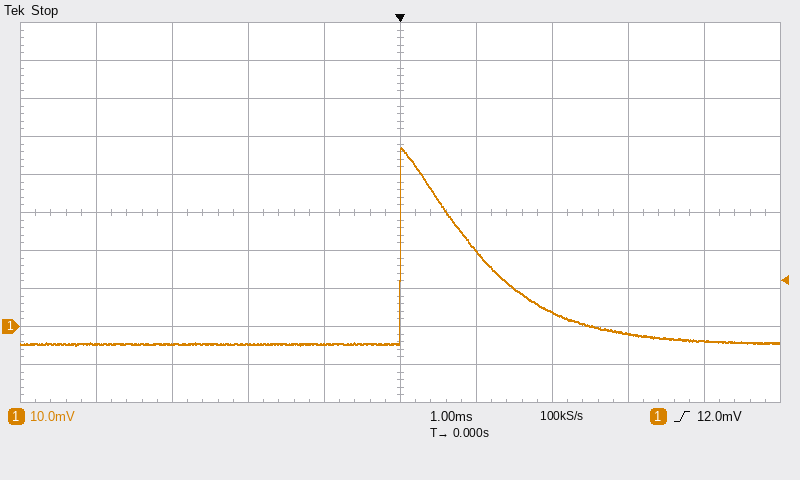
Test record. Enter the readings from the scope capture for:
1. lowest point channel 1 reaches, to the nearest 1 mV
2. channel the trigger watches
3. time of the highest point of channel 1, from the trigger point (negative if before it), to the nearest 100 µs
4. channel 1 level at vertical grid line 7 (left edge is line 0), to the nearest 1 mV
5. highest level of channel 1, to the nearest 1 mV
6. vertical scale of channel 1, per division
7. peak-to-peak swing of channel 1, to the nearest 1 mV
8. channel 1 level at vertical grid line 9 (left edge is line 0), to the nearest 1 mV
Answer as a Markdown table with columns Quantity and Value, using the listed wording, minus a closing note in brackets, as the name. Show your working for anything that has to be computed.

| Quantity | Value |
|---|---|
| lowest point channel 1 reaches, to the nearest 1 mV | -5 mV |
| channel the trigger watches | channel 1 |
| time of the highest point of channel 1, from the trigger point (negative if before it), to the nearest 100 µs | 0.0 ms |
| channel 1 level at vertical grid line 7 (left edge is line 0), to the nearest 1 mV | 4 mV |
| highest level of channel 1, to the nearest 1 mV | 47 mV |
| vertical scale of channel 1, per division | 10 mV |
| peak-to-peak swing of channel 1, to the nearest 1 mV | 47 mV − (-5 mV) = 52 mV |
| channel 1 level at vertical grid line 9 (left edge is line 0), to the nearest 1 mV | -4 mV |
